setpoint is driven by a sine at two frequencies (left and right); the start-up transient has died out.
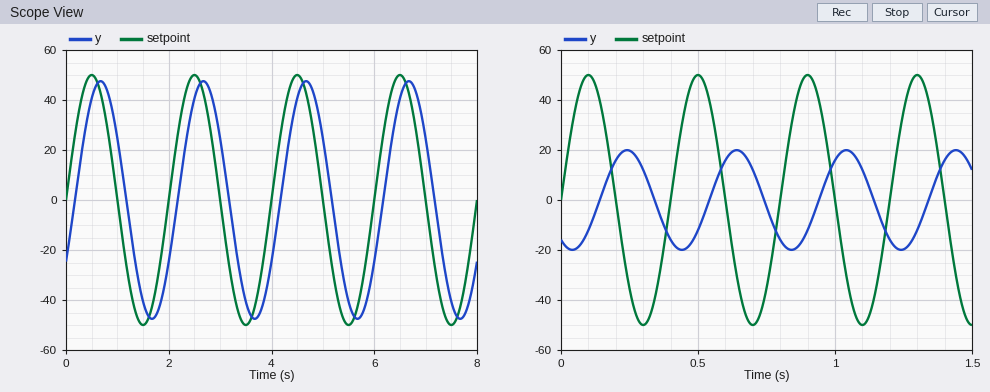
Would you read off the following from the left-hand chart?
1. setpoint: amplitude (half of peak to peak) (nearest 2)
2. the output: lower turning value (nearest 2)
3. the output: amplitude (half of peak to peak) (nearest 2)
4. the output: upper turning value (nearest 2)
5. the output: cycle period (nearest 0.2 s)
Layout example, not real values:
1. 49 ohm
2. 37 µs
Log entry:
1. 50
2. -48
3. 48
4. 48
5. 2.0 s
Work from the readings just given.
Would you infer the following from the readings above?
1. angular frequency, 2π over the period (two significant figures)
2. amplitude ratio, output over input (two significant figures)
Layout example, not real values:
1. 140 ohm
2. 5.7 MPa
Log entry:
1. 3.1 rad/s
2. 0.96
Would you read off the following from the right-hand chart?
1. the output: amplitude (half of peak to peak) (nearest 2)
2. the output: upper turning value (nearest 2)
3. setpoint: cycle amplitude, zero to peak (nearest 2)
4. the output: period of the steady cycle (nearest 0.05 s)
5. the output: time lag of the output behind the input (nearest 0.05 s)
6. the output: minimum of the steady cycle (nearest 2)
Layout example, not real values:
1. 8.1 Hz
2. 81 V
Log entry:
1. 20
2. 20
3. 50
4. 0.40 s
5. 0.15 s
6. -20
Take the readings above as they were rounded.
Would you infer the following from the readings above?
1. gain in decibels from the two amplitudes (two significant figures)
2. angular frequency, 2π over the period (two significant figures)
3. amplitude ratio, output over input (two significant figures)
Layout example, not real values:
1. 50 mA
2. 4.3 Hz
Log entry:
1. -8.0 dB
2. 16 rad/s
3. 0.40
